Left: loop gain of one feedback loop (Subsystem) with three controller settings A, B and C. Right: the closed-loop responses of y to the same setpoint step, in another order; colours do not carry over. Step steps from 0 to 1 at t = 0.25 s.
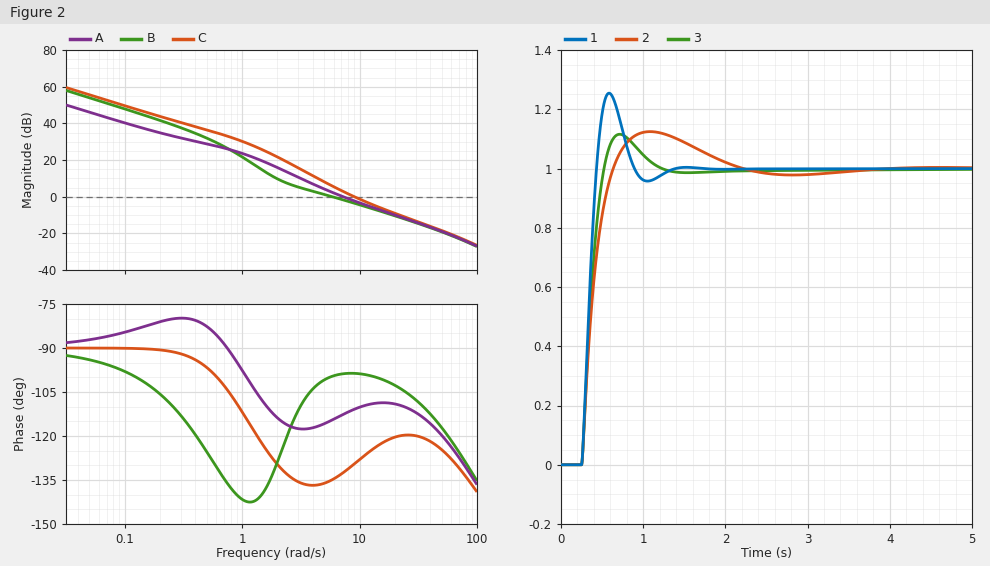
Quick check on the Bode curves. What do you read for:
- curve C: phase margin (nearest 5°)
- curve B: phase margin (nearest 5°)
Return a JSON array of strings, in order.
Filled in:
["50°", "80°"]
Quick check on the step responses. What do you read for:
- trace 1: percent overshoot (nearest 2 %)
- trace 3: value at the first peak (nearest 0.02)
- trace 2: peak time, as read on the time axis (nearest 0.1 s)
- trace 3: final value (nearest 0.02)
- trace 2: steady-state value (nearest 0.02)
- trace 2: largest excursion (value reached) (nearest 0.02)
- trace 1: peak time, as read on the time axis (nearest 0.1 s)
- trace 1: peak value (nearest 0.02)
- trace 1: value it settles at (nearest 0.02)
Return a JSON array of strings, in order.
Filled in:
["26 %", "1.12", "1.1 s", "1.00", "1.00", "1.12", "0.6 s", "1.26", "1.00"]
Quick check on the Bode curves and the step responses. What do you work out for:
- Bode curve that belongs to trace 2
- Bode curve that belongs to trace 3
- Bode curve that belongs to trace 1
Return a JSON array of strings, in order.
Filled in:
["B", "A", "C"]
